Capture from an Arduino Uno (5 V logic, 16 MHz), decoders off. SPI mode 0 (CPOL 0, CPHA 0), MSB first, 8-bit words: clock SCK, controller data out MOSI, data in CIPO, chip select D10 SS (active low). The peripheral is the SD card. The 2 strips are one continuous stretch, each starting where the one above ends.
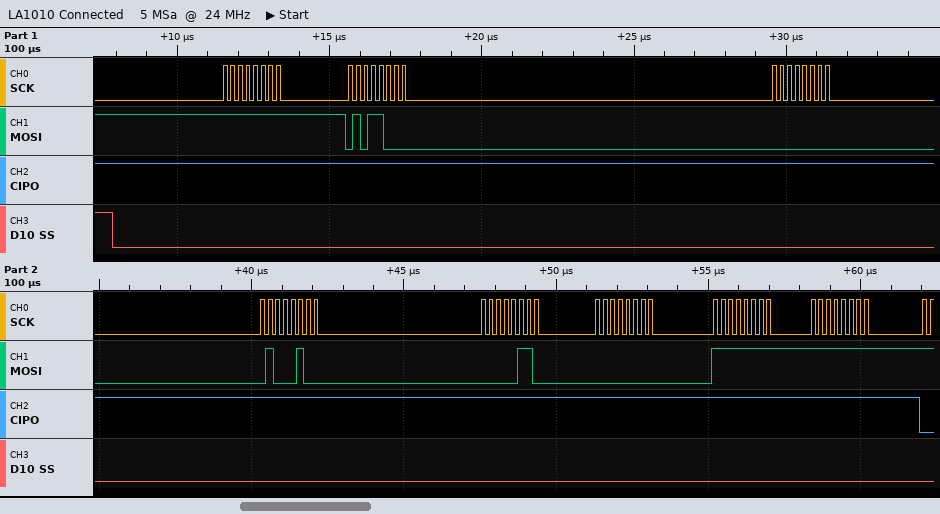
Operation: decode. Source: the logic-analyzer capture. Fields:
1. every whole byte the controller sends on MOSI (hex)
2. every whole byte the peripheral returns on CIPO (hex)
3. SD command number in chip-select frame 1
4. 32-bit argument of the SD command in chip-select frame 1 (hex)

0xFF 0x58 0x00 0x44 0x06 0x00 0xFF 0xFF
0xFF 0xFF 0xFF 0xFF 0xFF 0xFF 0xFF 0xFF
CMD24
0x00440600
